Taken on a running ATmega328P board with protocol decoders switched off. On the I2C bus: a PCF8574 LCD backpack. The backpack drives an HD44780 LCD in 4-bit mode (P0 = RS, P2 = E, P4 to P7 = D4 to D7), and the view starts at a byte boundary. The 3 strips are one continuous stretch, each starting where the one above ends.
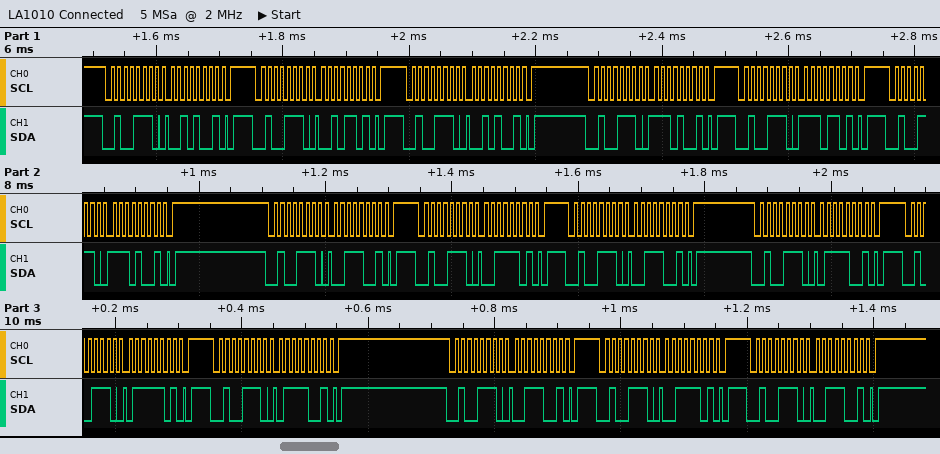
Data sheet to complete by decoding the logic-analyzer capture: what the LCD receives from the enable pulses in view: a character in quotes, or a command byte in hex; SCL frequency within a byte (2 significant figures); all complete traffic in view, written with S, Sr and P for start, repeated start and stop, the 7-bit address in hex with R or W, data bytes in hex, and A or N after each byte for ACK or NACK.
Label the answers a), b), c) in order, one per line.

a) '.' '7'
b) 100 kHz
c) S 27W A 29 A P S 27W A 2D A P S 27W A 29 A P S 27W A E9 A P S 27W A ED A P S 27W A E9 A P S 27W A 39 A P S 27W A 3D A P S 27W A 39 A P S 27W A 79 A P S 27W A 7D A P S 27W A 79 A P S 27W A 39 A P S 27W A 3D A P S 27W A 39 A P
